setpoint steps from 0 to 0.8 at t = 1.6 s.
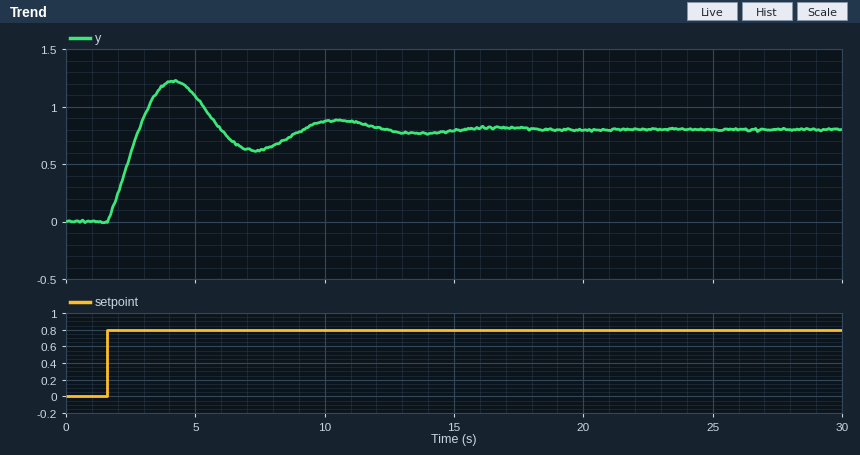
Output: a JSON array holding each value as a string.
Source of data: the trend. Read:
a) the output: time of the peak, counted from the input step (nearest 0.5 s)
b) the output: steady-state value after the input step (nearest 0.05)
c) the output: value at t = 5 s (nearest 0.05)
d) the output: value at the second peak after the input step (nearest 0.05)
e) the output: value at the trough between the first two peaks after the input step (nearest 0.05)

["2.5 s", "0.80", "1.10", "0.90", "0.60"]
